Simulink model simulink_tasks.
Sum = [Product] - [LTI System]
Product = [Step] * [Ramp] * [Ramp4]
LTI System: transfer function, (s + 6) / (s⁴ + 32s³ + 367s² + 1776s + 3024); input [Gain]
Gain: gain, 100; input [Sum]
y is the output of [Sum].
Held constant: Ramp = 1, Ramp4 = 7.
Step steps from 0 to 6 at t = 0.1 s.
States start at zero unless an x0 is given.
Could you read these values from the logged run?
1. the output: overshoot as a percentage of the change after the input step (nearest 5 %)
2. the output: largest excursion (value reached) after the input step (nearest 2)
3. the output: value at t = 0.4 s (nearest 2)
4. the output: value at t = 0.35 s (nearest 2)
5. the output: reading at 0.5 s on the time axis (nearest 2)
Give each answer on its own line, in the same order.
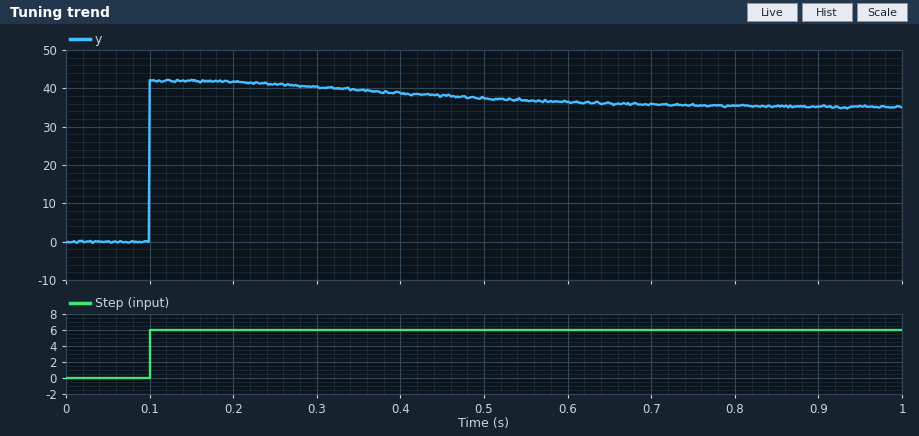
20 %
42
38
40
38
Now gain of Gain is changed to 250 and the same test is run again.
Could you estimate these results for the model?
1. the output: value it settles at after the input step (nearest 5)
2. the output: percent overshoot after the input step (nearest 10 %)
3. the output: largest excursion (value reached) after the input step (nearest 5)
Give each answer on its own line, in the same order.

30
50 %
40
